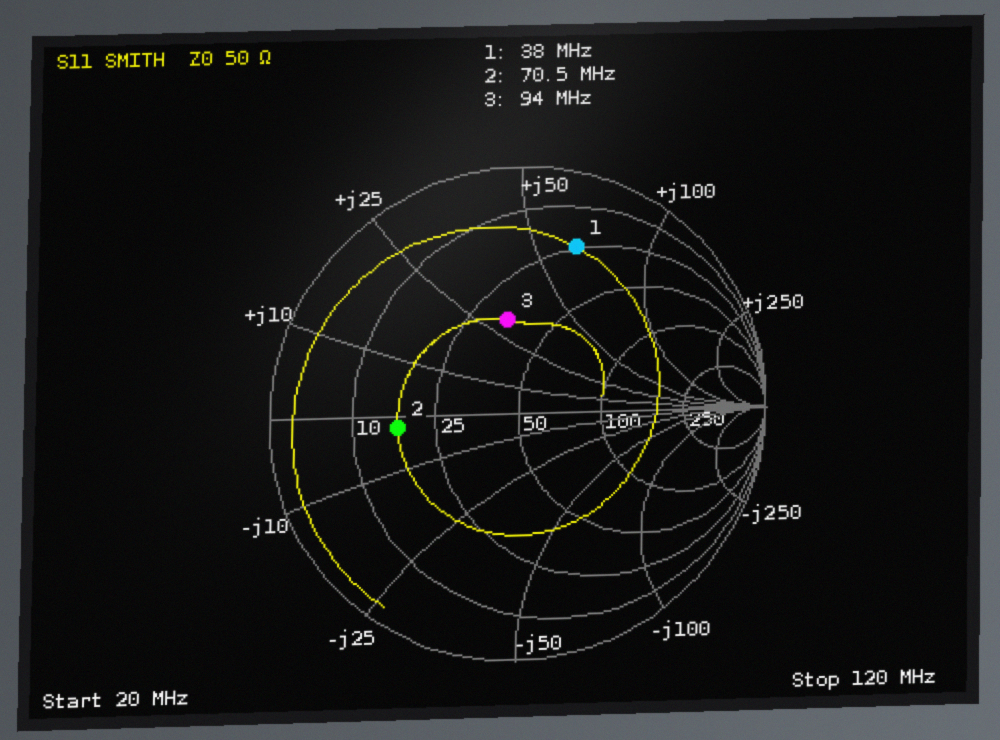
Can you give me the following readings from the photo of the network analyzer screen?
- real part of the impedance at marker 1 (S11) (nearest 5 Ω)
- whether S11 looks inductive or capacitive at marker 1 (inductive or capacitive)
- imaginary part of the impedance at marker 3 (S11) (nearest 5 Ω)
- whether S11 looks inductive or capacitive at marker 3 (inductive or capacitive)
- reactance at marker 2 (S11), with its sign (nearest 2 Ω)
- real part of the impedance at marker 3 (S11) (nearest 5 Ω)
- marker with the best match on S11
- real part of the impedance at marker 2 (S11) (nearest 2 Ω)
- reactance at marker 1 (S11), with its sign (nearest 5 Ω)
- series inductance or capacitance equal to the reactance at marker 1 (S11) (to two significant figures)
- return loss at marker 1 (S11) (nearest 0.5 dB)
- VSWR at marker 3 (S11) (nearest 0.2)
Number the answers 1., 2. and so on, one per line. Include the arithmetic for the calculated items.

1. 25 Ω
2. inductive
3. +30 Ω
4. inductive
5. -2 Ω
6. 35 Ω
7. marker 3
8. 18 Ω
9. +65 Ω
10. L = 65 Ω/(2π × 38 MHz) ≈ 272 nH, so 270 nH to two significant figures
11. 3.0 dB
12. 2.2
